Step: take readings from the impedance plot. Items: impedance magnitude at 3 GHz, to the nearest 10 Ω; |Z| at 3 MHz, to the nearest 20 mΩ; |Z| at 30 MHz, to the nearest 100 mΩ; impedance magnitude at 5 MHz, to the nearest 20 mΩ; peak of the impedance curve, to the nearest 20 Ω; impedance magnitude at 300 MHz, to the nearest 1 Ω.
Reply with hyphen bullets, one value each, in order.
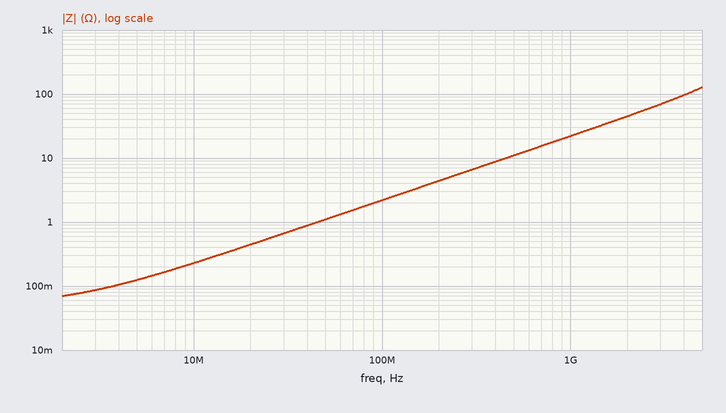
- 70 Ω
- 80 mΩ
- 700 mΩ
- 120 mΩ
- 120 Ω
- 7 Ω
